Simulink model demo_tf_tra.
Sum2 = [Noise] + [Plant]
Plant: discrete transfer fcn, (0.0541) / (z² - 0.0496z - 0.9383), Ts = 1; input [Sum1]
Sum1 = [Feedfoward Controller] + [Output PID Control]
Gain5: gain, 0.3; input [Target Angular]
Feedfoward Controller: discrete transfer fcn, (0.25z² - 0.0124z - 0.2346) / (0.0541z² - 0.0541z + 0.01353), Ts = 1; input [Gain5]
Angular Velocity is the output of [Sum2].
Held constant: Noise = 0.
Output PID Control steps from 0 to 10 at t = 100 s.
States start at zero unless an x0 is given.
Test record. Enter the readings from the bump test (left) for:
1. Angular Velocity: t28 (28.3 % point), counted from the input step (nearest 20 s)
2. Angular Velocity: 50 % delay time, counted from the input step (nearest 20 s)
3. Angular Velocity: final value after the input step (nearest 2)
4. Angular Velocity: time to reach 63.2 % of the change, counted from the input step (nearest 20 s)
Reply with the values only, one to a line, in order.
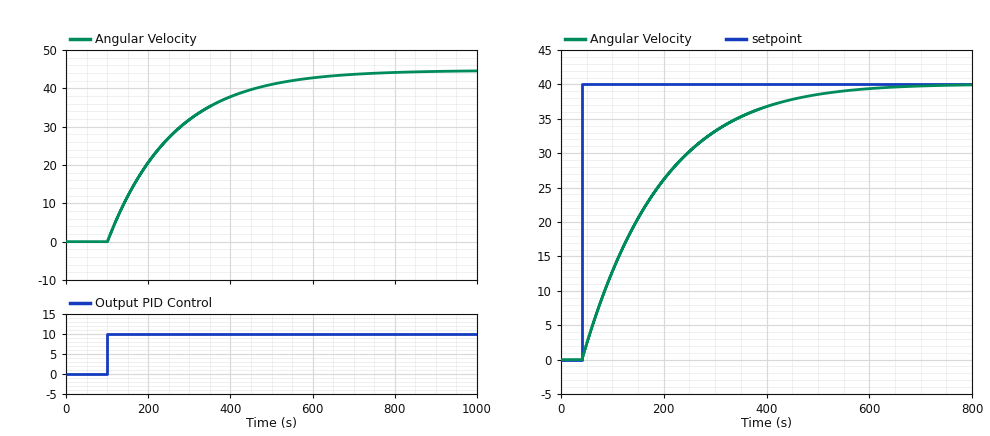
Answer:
60 s
120 s
44
160 s
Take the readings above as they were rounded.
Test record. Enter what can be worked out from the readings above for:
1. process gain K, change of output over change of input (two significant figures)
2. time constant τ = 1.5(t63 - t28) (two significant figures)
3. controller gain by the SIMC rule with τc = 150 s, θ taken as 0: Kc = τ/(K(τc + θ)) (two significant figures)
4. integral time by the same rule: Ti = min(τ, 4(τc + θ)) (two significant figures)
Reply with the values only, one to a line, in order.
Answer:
4.4
150 s
0.23
150 s
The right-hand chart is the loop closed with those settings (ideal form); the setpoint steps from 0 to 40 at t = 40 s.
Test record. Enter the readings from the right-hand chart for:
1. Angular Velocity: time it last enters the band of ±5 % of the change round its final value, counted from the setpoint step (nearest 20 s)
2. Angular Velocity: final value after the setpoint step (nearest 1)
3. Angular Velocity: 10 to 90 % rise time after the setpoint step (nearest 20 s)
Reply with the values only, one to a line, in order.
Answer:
420 s
40
320 s
